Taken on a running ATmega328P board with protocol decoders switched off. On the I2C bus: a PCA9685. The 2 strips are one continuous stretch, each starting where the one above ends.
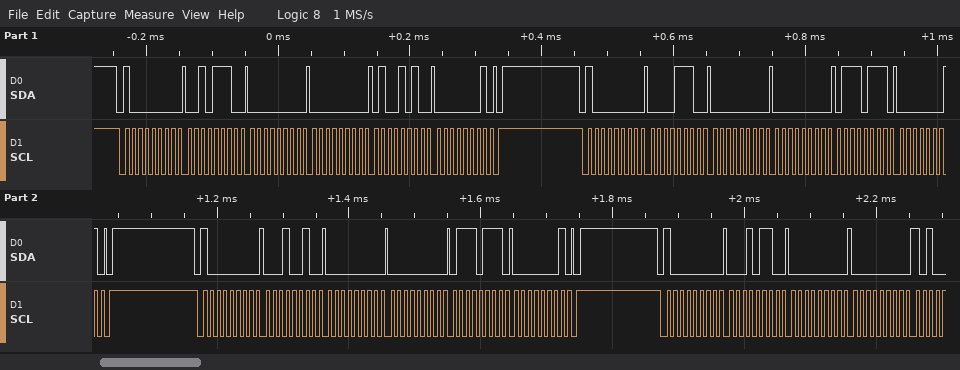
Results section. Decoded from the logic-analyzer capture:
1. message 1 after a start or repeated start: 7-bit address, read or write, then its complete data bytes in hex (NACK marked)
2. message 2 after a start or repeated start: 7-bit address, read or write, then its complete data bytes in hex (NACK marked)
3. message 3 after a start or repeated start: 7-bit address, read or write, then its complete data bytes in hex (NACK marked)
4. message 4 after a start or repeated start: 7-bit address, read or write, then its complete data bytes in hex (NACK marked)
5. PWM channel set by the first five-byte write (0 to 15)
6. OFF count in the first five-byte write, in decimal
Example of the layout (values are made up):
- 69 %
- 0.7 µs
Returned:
- 0x40 write: 2E 00 00 4A 01
- 0x40 write: 0E 00 00 77 01
- 0x40 write: 12 00 00 77 01
- 0x40 write: 16 00 00
- 10
- 330
